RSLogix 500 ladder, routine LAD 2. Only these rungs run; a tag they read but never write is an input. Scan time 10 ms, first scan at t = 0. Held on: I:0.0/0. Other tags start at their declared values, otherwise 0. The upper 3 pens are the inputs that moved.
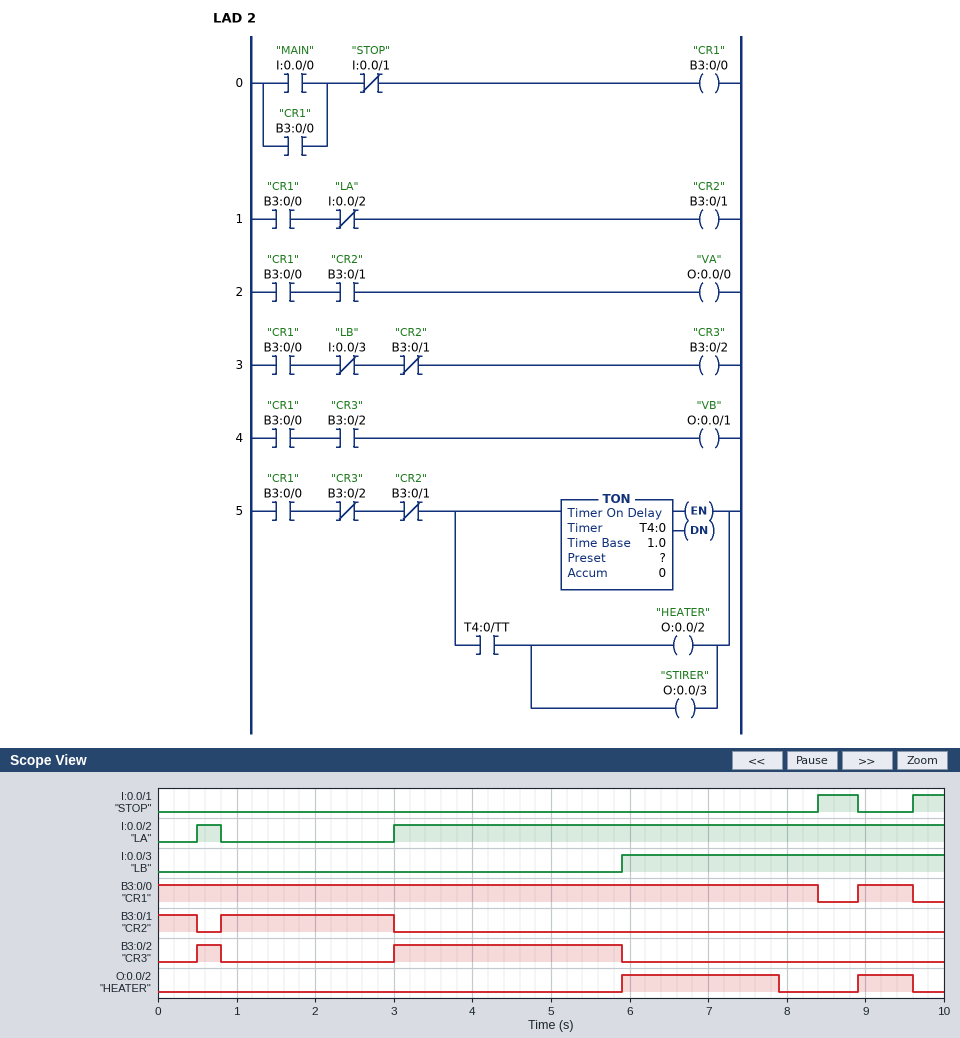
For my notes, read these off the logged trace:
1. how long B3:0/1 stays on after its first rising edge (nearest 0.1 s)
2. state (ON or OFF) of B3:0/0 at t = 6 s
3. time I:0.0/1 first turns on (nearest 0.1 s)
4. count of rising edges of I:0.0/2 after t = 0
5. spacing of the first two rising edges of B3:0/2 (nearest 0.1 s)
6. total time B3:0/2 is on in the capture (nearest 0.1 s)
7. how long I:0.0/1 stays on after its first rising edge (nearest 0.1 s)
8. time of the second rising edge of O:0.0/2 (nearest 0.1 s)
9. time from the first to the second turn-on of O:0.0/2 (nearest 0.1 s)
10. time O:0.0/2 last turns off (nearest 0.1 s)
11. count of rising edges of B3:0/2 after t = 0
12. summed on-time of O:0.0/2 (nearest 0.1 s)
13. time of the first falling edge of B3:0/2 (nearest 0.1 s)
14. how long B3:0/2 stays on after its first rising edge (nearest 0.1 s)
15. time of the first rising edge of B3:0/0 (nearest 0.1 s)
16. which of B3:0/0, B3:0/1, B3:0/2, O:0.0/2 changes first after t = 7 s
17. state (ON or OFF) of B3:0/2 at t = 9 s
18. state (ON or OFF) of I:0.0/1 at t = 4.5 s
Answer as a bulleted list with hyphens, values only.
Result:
- 2.2 s
- ON
- 8.4 s
- 2
- 2.5 s
- 3.2 s
- 0.5 s
- 8.9 s
- 3.0 s
- 9.6 s
- 2
- 2.7 s
- 0.8 s
- 0.3 s
- 8.9 s
- O:0.0/2
- OFF
- OFF
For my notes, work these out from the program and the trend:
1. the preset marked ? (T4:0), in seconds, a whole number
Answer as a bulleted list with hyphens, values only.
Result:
- 2 s
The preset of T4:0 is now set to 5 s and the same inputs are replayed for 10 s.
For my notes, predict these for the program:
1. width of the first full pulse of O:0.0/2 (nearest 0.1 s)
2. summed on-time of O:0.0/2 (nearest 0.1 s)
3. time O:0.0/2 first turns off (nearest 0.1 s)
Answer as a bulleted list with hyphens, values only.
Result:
- 2.5 s
- 3.2 s
- 8.4 s
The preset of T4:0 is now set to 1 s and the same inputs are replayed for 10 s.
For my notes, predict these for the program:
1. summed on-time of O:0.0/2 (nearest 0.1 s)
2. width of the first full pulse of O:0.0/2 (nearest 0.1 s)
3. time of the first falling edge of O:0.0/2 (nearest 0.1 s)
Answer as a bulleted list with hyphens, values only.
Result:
- 1.7 s
- 1.0 s
- 6.9 s
